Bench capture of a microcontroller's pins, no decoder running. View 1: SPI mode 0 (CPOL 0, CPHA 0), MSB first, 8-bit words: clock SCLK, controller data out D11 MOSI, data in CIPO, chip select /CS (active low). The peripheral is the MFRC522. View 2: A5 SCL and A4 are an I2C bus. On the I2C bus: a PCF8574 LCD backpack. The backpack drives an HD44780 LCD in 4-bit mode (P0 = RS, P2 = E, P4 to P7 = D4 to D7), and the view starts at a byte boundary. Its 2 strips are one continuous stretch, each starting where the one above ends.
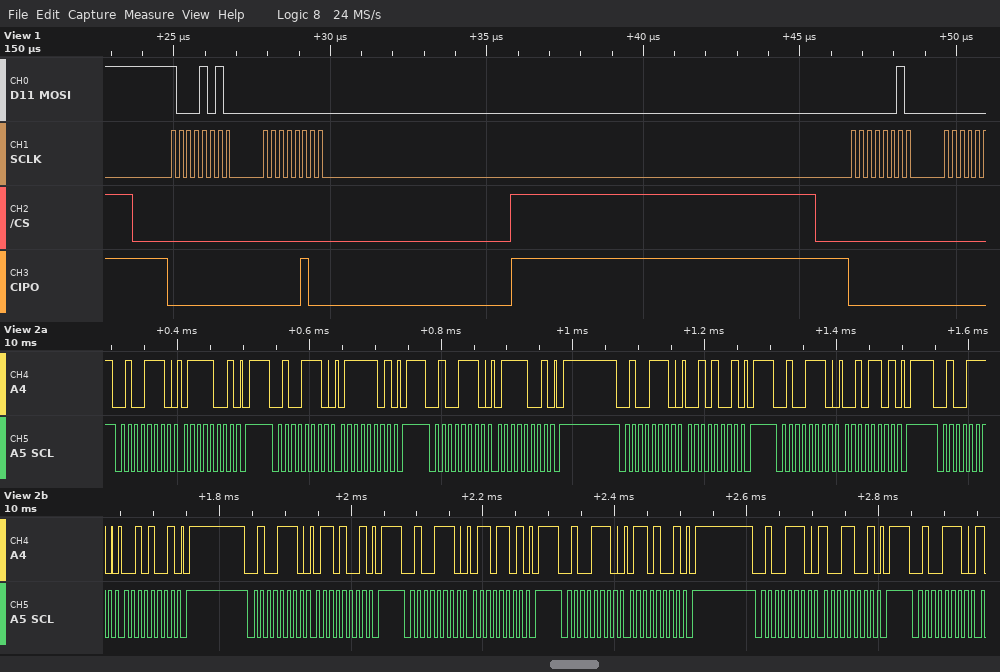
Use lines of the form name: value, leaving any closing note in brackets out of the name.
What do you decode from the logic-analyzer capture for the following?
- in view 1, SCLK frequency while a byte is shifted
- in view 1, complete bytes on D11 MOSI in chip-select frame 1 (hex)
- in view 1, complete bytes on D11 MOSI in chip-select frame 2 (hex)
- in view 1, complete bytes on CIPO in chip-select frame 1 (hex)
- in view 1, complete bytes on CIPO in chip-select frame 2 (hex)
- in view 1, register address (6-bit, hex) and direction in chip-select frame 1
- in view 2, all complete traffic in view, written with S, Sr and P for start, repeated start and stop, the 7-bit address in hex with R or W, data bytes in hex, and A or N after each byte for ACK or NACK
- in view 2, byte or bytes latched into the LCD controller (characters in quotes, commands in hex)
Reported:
in view 1, SCLK frequency while a byte is shifted: 4 MHz
in view 1, complete bytes on D11 MOSI in chip-select frame 1: 8A 00
in view 1, complete bytes on D11 MOSI in chip-select frame 2: 02
in view 1, complete bytes on CIPO in chip-select frame 1: 00 04
in view 1, complete bytes on CIPO in chip-select frame 2: 00
in view 1, register address (6-bit, hex) and direction in chip-select frame 1: 0x05 read
in view 2, all complete traffic in view, written with S, Sr and P for start, repeated start and stop, the 7-bit address in hex with R or W, data bytes in hex, and A or N after each byte for ACK or NACK: S 27W A 79 A P S 27W A 7D A P S 27W A 79 A P S 27W A 29 A P S 27W A 2D A P S 27W A 29 A P S 27W A 69 A P S 27W A 6D A P S 27W A 69 A P S 27W A 99 A P S 27W A
in view 2, byte or bytes latched into the LCD controller: 'r'
